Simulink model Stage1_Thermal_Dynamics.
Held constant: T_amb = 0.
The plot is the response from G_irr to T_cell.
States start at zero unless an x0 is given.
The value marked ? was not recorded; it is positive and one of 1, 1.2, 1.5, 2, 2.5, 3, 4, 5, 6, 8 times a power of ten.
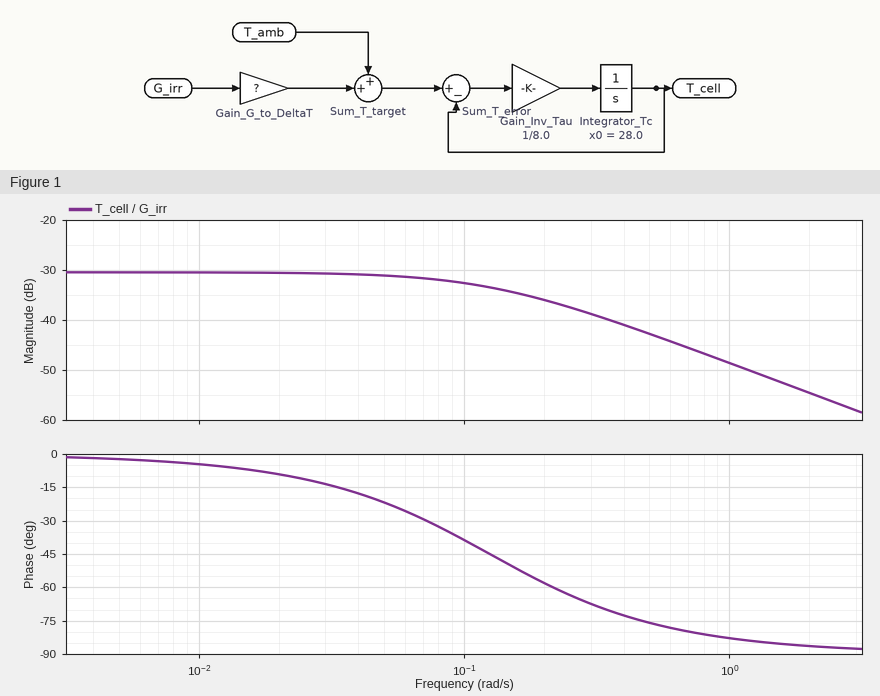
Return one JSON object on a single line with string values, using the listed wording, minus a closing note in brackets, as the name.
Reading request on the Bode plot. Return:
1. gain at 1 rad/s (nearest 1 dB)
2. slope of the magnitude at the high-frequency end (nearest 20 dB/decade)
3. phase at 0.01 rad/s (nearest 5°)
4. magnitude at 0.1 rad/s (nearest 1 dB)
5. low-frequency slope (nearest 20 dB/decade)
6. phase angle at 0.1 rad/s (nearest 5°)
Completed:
{"gain at 1 rad/s": "-49 dB", "slope of the magnitude at the high-frequency end": "-20 dB/decade", "phase at 0.01 rad/s": "-5°", "magnitude at 0.1 rad/s": "-33 dB", "low-frequency slope": "0 dB/decade", "phase angle at 0.1 rad/s": "-40°"}
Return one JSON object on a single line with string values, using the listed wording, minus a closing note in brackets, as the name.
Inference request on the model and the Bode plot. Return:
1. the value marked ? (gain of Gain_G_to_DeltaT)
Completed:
{"the value marked ?": "0.03"}
